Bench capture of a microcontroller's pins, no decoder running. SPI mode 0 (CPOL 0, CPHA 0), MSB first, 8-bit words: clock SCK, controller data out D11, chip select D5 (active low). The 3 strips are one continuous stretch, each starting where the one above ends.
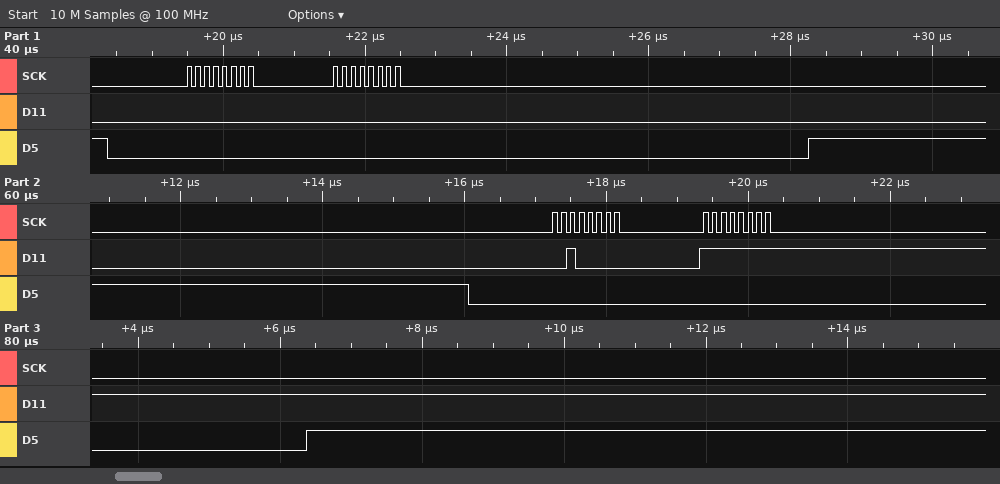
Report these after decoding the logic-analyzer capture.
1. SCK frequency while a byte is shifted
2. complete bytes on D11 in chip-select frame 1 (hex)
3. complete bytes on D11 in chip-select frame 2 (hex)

8 MHz
0x00 0x00
0x20 0xFF
